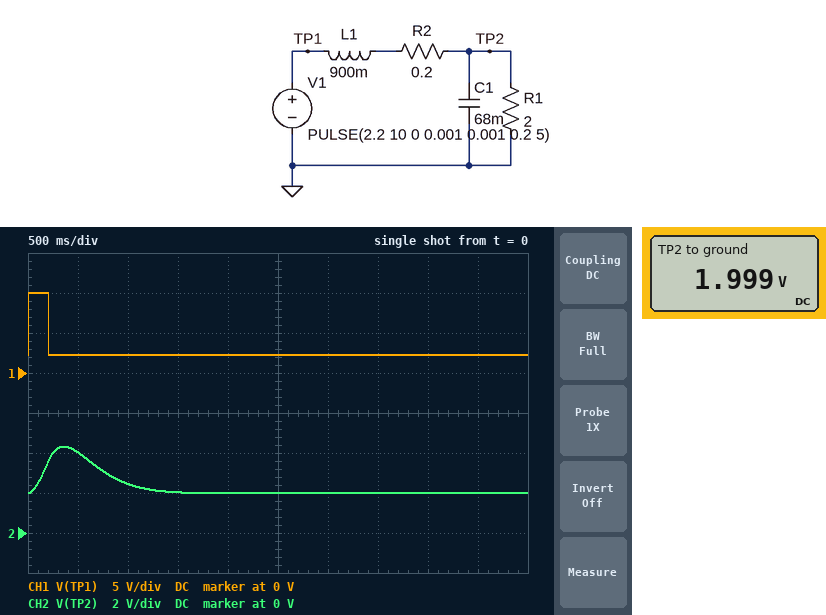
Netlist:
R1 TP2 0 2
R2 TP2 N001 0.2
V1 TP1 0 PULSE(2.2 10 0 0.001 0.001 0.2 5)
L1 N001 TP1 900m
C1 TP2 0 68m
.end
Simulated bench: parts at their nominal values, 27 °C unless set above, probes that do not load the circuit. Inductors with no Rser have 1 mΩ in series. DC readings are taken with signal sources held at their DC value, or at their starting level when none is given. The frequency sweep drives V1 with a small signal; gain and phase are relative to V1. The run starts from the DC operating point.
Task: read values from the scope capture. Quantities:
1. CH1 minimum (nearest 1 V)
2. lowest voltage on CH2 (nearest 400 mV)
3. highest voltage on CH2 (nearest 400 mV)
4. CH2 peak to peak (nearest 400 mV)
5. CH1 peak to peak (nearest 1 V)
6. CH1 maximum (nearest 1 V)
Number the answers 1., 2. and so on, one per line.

1. 2 V
2. 2.0 V
3. 4.4 V
4. 2.4 V
5. 8 V
6. 10 V
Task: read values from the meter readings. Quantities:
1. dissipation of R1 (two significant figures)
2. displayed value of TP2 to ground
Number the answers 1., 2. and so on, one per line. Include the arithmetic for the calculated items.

1. (1.999 V)^2 / 2 Ω = 2.0 W
2. 1.999 V
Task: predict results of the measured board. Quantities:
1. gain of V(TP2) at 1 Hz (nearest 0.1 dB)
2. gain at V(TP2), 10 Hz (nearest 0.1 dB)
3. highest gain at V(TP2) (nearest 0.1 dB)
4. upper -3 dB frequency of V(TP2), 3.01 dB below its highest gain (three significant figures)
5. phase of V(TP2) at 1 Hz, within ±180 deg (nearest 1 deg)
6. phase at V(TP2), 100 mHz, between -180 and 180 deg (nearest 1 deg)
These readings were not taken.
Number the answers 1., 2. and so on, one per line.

1. -10.1 dB
2. -47.7 dB
3. -0.8 dB
4. 509 mHz
5. -114 deg
6. -15 deg
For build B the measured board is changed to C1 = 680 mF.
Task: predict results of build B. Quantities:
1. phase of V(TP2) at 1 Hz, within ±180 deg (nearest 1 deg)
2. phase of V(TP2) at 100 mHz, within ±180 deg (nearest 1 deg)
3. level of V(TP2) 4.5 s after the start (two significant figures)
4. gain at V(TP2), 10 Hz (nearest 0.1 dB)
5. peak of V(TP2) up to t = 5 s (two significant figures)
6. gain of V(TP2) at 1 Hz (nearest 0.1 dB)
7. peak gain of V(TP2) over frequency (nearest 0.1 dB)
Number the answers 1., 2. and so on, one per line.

1. -171 deg
2. -23 deg
3. 1.8 V
4. -67.7 dB
5. 3.2 V
6. -27.4 dB
7. 2.7 dB
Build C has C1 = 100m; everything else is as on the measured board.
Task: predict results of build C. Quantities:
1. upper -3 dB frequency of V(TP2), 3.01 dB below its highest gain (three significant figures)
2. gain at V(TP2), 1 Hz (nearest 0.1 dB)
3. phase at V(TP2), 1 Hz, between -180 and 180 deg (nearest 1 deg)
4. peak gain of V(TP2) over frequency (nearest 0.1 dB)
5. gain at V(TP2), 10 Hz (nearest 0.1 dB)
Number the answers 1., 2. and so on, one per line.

1. 525 mHz
2. -11.7 dB
3. -130 deg
4. -0.8 dB
5. -51.0 dB
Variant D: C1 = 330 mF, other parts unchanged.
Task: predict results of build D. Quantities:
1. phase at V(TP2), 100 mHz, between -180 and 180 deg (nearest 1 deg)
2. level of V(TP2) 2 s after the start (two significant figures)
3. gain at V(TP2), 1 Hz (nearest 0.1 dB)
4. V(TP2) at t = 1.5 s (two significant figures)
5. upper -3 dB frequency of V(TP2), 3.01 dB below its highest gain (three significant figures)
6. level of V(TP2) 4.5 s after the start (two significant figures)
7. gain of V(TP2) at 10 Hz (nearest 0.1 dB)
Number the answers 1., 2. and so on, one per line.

1. -18 deg
2. 1.9 V
3. -20.9 dB
4. 2.6 V
5. 362 mHz
6. 2.1 V
7. -61.4 dB
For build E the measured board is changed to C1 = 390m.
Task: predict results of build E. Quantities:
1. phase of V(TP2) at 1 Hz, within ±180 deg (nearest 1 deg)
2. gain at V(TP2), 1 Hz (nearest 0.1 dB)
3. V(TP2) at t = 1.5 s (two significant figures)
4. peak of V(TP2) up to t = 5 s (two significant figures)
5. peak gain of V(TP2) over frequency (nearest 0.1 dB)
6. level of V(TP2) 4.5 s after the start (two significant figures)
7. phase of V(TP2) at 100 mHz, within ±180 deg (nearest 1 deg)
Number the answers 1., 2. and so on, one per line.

1. -165 deg
2. -22.4 dB
3. 2.8 V
4. 3.5 V
5. 1.4 dB
6. 2.1 V
7. -19 deg
